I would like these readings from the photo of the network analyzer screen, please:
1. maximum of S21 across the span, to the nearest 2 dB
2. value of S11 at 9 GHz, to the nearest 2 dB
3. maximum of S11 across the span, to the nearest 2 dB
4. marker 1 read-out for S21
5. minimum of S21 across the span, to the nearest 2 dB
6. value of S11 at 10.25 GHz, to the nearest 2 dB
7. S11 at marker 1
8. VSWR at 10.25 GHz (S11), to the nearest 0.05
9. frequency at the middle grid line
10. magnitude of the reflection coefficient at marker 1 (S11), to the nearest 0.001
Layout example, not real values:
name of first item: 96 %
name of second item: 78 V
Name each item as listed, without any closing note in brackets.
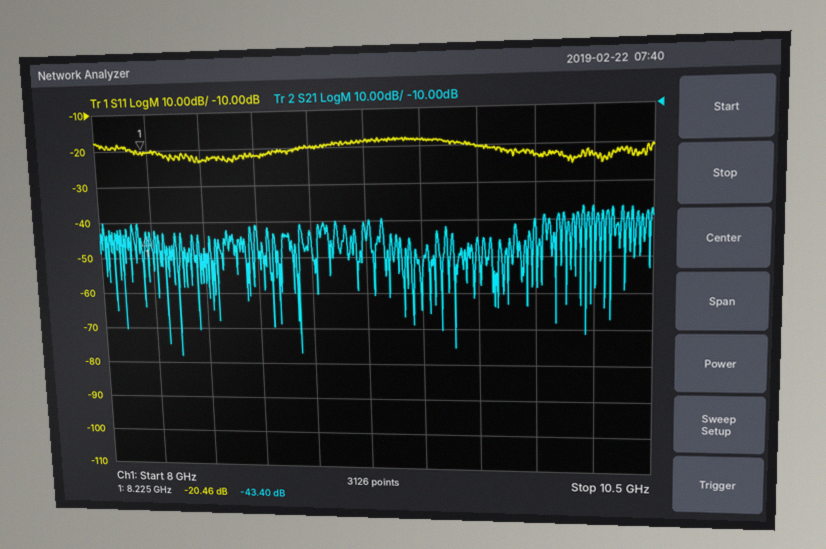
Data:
maximum of S21 across the span, to the nearest 2 dB: -36 dB
value of S11 at 9 GHz, to the nearest 2 dB: -20 dB
maximum of S11 across the span, to the nearest 2 dB: -18 dB
marker 1 read-out for S21: -43.40 dB
minimum of S21 across the span, to the nearest 2 dB: -78 dB
value of S11 at 10.25 GHz, to the nearest 2 dB: -24 dB
S11 at marker 1: -20.46 dB
VSWR at 10.25 GHz (S11), to the nearest 0.05: 1.15
frequency at the middle grid line: 9.25 GHz
magnitude of the reflection coefficient at marker 1 (S11), to the nearest 0.001: 0.095
